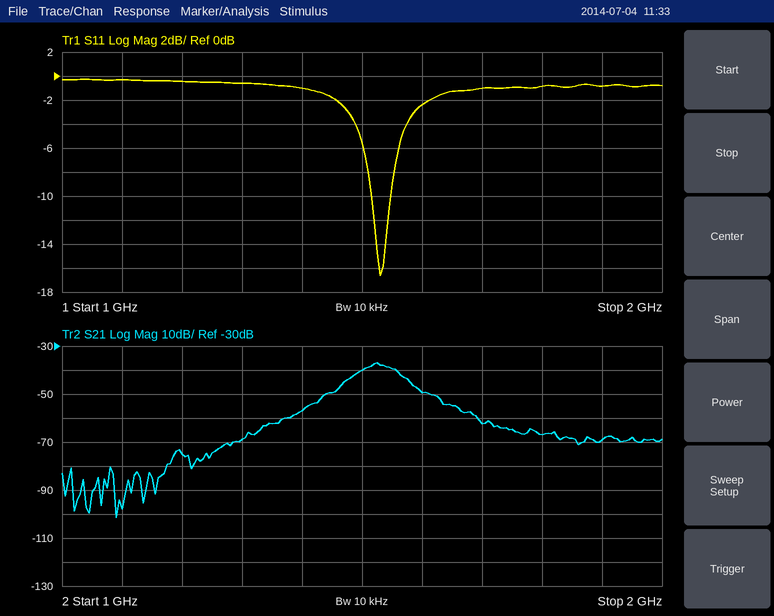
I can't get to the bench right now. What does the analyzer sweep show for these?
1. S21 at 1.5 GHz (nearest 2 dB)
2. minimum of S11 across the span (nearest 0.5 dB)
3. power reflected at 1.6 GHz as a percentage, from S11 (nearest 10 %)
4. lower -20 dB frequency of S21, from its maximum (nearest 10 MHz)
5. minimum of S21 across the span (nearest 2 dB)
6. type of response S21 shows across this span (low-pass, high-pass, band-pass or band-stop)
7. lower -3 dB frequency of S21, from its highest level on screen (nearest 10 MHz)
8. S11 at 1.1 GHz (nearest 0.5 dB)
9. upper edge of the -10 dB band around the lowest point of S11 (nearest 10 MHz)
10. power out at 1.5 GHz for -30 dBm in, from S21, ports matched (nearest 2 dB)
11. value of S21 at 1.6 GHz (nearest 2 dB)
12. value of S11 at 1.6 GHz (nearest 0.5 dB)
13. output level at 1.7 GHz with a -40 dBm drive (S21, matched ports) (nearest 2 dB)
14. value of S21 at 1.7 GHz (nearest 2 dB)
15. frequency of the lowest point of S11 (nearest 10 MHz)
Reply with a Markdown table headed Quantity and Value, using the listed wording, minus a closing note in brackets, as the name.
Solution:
| Quantity | Value |
|---|---|
| S21 at 1.5 GHz | -40 dB |
| minimum of S11 across the span | -16.5 dB |
| power reflected at 1.6 GHz as a percentage, from S11 | 60 % |
| lower -20 dB frequency of S21, from its maximum | 1.40 GHz |
| minimum of S21 across the span | -102 dB |
| type of response S21 shows across this span | band-pass |
| lower -3 dB frequency of S21, from its highest level on screen | 1.50 GHz |
| S11 at 1.1 GHz | -0.5 dB |
| upper edge of the -10 dB band around the lowest point of S11 | 1.55 GHz |
| power out at 1.5 GHz for -30 dBm in, from S21, ports matched | -70 dBm |
| value of S21 at 1.6 GHz | -50 dB |
| value of S11 at 1.6 GHz | -2.5 dB |
| output level at 1.7 GHz with a -40 dBm drive (S21, matched ports) | -102 dBm |
| value of S21 at 1.7 GHz | -62 dB |
| frequency of the lowest point of S11 | 1.53 GHz |
